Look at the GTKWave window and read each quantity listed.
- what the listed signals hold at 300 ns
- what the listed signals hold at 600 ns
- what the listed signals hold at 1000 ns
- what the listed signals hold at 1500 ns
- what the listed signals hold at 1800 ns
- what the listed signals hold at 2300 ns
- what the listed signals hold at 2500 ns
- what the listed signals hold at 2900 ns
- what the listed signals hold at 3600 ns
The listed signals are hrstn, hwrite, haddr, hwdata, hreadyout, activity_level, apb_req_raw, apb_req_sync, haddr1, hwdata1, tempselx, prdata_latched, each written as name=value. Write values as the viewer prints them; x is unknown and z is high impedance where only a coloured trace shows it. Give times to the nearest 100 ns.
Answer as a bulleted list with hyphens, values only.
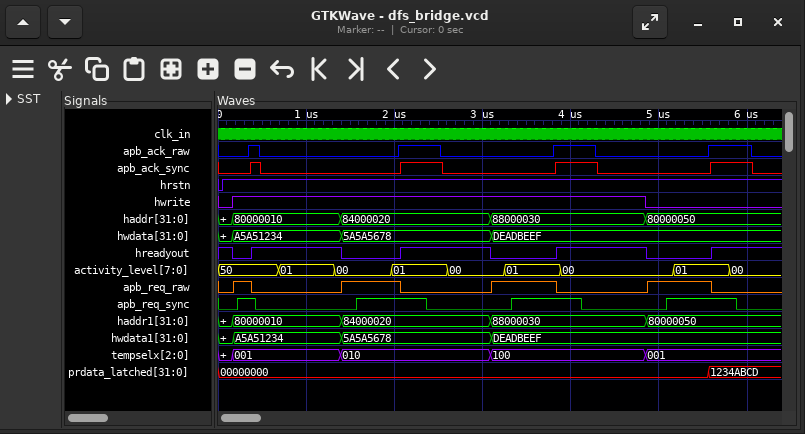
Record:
- hrstn=1, hwrite=1, haddr=80000010, hwdata=A5A51234, hreadyout=0, activity_level=50, apb_req_raw=1, apb_req_sync=1, haddr1=80000010, hwdata1=A5A51234, tempselx=001, prdata_latched=00000000
- hrstn=1, hwrite=1, haddr=80000010, hwdata=A5A51234, hreadyout=1, activity_level=50, apb_req_raw=0, apb_req_sync=0, haddr1=80000010, hwdata1=A5A51234, tempselx=001, prdata_latched=00000000
- hrstn=1, hwrite=1, haddr=80000010, hwdata=A5A51234, hreadyout=1, activity_level=01, apb_req_raw=0, apb_req_sync=0, haddr1=80000010, hwdata1=A5A51234, tempselx=001, prdata_latched=00000000
- hrstn=1, hwrite=1, haddr=84000020, hwdata=5A5A5678, hreadyout=0, activity_level=00, apb_req_raw=1, apb_req_sync=0, haddr1=84000020, hwdata1=5A5A5678, tempselx=010, prdata_latched=00000000
- hrstn=1, hwrite=1, haddr=84000020, hwdata=5A5A5678, hreadyout=0, activity_level=00, apb_req_raw=1, apb_req_sync=1, haddr1=84000020, hwdata1=5A5A5678, tempselx=010, prdata_latched=00000000
- hrstn=1, hwrite=1, haddr=84000020, hwdata=5A5A5678, hreadyout=1, activity_level=01, apb_req_raw=0, apb_req_sync=1, haddr1=84000020, hwdata1=5A5A5678, tempselx=010, prdata_latched=00000000
- hrstn=1, hwrite=1, haddr=84000020, hwdata=5A5A5678, hreadyout=1, activity_level=01, apb_req_raw=0, apb_req_sync=0, haddr1=84000020, hwdata1=5A5A5678, tempselx=010, prdata_latched=00000000
- hrstn=1, hwrite=1, haddr=84000020, hwdata=5A5A5678, hreadyout=1, activity_level=00, apb_req_raw=0, apb_req_sync=0, haddr1=84000020, hwdata1=5A5A5678, tempselx=010, prdata_latched=00000000
- hrstn=1, hwrite=1, haddr=88000030, hwdata=DEADBEEF, hreadyout=0, activity_level=01, apb_req_raw=1, apb_req_sync=1, haddr1=88000030, hwdata1=DEADBEEF, tempselx=100, prdata_latched=00000000
